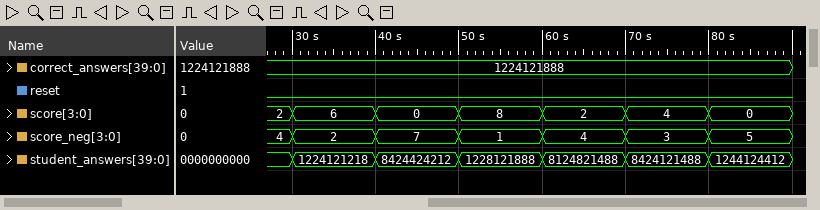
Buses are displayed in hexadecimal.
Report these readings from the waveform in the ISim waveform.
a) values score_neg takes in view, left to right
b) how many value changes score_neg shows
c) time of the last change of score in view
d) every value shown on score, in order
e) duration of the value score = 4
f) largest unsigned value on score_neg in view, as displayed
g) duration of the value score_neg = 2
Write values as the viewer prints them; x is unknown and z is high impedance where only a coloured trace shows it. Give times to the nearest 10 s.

4, 2, 7, 1, 4, 3, 5
6
80 s
2, 6, 0, 8, 2, 4, 0
10 s
7
10 s
